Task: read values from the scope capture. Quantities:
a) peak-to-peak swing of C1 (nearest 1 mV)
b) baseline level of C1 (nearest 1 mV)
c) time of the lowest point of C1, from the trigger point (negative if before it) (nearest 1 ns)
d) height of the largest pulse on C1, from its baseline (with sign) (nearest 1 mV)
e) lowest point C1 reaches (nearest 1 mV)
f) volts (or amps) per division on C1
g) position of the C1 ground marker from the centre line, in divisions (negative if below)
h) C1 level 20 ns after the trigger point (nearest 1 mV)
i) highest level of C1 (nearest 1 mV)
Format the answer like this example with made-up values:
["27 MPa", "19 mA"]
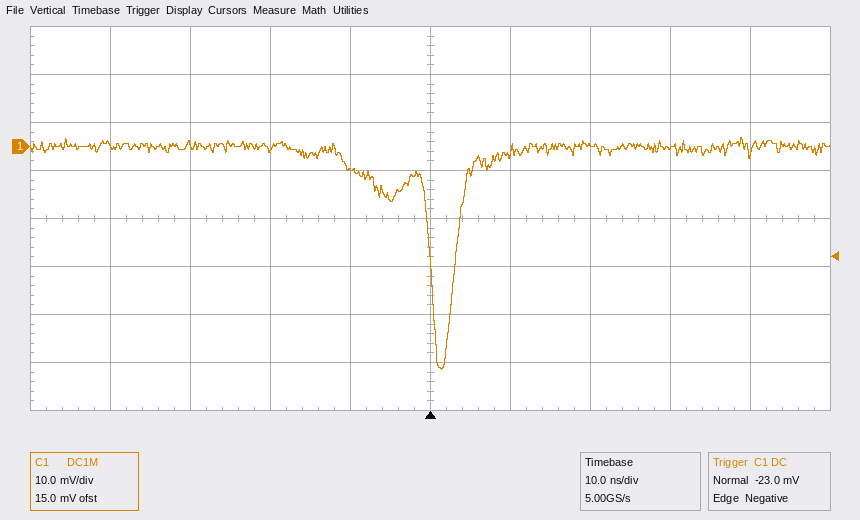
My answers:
["48 mV", "0 mV", "+1 ns", "-46 mV", "-46 mV", "10 mV", "+1.5 div", "0 mV", "2 mV"]
